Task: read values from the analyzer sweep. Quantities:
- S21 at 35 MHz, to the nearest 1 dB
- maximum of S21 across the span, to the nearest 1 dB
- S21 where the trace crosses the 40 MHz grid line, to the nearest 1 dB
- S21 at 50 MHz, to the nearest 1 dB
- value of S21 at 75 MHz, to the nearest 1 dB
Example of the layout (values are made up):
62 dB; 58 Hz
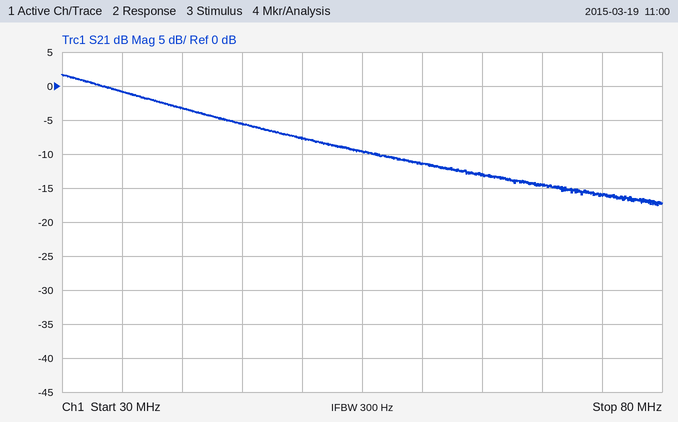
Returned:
-1 dB; 2 dB; -3 dB; -8 dB; -16 dB
